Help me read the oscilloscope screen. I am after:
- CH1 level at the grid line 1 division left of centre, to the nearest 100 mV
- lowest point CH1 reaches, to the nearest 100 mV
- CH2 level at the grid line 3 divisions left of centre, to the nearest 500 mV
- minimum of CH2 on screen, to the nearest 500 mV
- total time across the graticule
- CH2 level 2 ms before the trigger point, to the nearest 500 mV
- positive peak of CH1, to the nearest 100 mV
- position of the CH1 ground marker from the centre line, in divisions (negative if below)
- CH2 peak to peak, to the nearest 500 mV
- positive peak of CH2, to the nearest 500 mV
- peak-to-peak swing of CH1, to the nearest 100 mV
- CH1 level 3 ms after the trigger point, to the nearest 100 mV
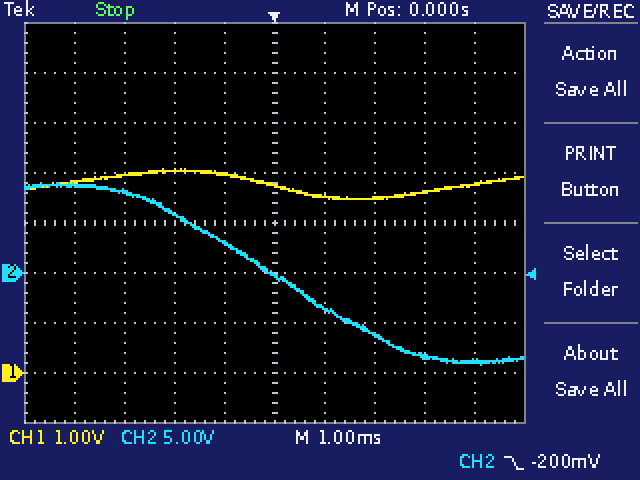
4.0 V
3.5 V
8.0 V
-9.0 V
10 ms
6.0 V
4.1 V
-3.0 div
18.0 V
9.0 V
600 mV
3.6 V
